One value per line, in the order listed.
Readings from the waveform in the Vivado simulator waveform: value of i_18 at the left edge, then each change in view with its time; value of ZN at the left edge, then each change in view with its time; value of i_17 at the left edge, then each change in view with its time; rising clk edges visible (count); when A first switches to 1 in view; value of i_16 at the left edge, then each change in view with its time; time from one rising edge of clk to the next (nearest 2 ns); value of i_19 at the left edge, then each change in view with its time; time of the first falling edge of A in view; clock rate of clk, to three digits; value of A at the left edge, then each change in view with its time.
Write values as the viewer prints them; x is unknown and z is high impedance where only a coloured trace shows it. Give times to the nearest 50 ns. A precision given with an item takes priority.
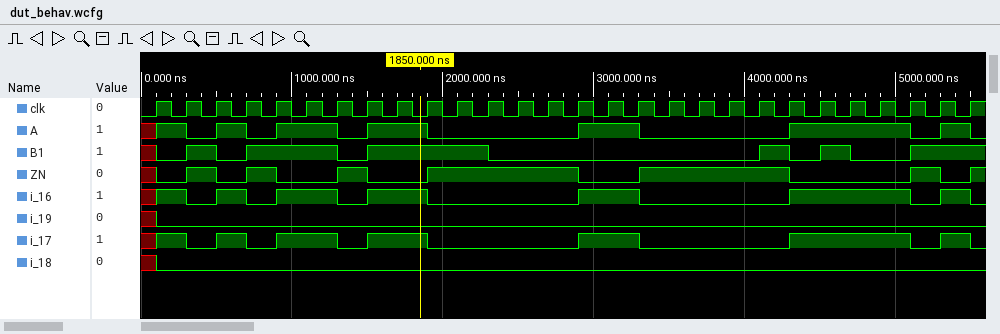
x, 0 at 100 ns
x, 0 at 100 ns, 1 at 300 ns, 0 at 500 ns, 1 at 700 ns, 0 at 900 ns, 1 at 1300 ns, 0 at 1500 ns, 1 at 1900 ns, 0 at 2900 ns, 1 at 3300 ns, 0 at 4300 ns, 1 at 5100 ns, 0 at 5300 ns, 1 at 5500 ns
x, 1 at 100 ns, 0 at 300 ns, 1 at 500 ns, 0 at 700 ns, 1 at 900 ns, 0 at 1300 ns, 1 at 1500 ns, 0 at 1900 ns, 1 at 2900 ns, 0 at 3300 ns, 1 at 4300 ns, 0 at 5100 ns, 1 at 5300 ns, 0 at 5500 ns
28
100 ns
x, 1 at 100 ns, 0 at 300 ns, 1 at 500 ns, 0 at 700 ns, 1 at 900 ns, 0 at 1300 ns, 1 at 1500 ns, 0 at 1900 ns, 1 at 2900 ns, 0 at 3300 ns, 1 at 4300 ns, 0 at 5100 ns, 1 at 5300 ns, 0 at 5500 ns
200 ns
x, 0 at 100 ns
300 ns
5.00 MHz
x, 1 at 100 ns, 0 at 300 ns, 1 at 500 ns, 0 at 700 ns, 1 at 900 ns, 0 at 1300 ns, 1 at 1500 ns, 0 at 1900 ns, 1 at 2900 ns, 0 at 3300 ns, 1 at 4300 ns, 0 at 5100 ns, 1 at 5300 ns, 0 at 5500 ns
